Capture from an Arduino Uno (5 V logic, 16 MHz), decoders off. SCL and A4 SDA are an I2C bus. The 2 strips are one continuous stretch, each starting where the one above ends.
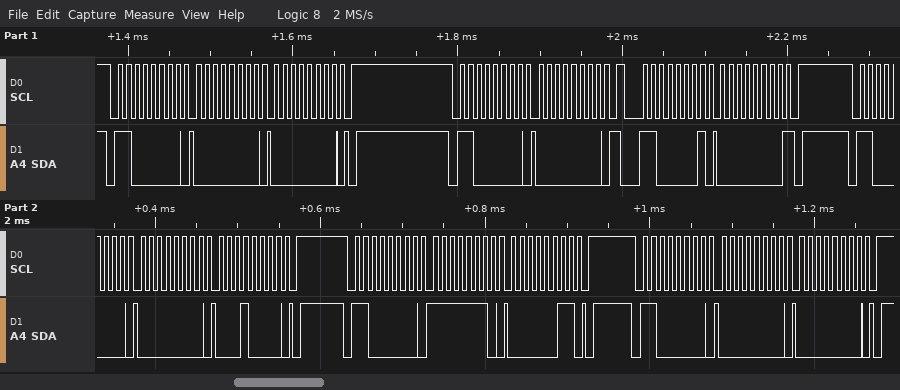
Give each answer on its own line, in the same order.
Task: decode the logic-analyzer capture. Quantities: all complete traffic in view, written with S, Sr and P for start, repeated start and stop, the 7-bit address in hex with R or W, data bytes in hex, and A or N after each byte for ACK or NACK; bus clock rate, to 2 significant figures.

S 60W A 00 A 00 A P S 60W A 00 A Sr 60R A 00 N P S 60W A 00 A 10 A P S 60W A FE A 03 A P S 60W A 00 A 00 A P
100 kHz
